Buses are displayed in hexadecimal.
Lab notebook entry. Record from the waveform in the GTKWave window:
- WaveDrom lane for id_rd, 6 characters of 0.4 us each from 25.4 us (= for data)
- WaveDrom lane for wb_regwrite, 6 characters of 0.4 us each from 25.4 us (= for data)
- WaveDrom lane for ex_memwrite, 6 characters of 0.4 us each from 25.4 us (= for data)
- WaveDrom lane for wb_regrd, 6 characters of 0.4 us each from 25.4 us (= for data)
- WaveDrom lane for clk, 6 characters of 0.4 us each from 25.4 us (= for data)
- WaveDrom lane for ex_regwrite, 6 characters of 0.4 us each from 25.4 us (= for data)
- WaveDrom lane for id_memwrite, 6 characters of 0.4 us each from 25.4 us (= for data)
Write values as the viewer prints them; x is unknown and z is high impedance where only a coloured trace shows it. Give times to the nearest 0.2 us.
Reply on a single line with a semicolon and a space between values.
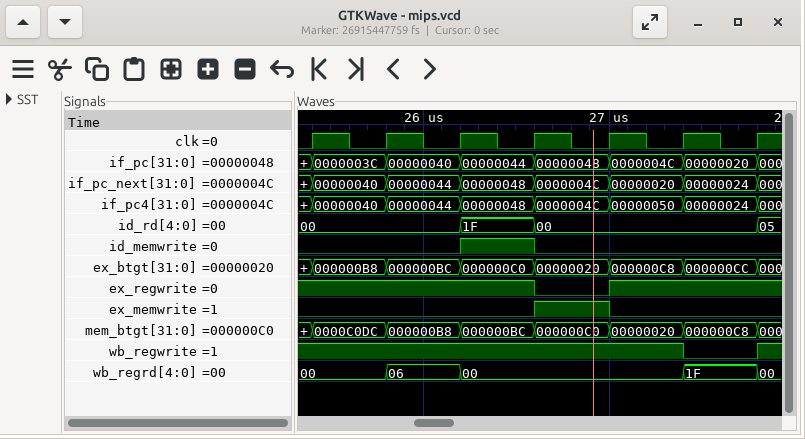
{name: 'id_rd', wave: '=.==..', data: '00 1F 00'}; {name: 'wb_regwrite', wave: '1....0'}; {name: 'ex_memwrite', wave: '0..10.'}; {name: 'wb_regrd', wave: '===..=', data: '00 06 00 1F'}; {name: 'clk', wave: 'p.....'}; {name: 'ex_regwrite', wave: '1..01.'}; {name: 'id_memwrite', wave: '0.10..'}
